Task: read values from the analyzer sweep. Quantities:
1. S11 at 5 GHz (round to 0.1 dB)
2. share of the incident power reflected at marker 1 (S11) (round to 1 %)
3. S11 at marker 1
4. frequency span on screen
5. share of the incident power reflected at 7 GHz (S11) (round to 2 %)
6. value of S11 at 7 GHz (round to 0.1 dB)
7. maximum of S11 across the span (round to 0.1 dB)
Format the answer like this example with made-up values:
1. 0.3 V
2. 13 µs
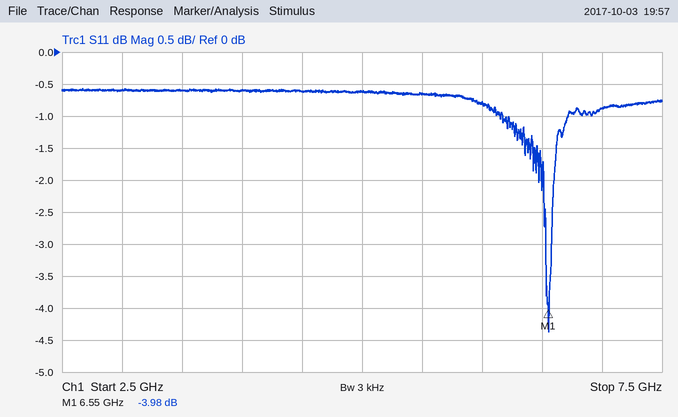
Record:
1. -0.6 dB
2. 40 %
3. -3.98 dB
4. 5 GHz
5. 82 %
6. -0.9 dB
7. -0.6 dB
